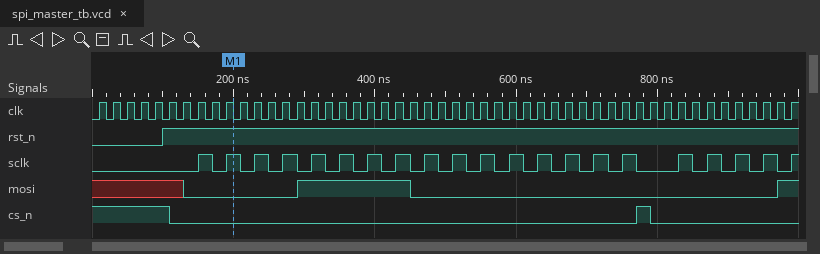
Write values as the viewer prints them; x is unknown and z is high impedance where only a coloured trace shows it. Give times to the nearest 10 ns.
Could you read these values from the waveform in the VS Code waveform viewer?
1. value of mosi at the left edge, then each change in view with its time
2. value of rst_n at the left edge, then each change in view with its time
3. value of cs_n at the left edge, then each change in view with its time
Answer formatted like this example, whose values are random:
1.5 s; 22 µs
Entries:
x, 0 at 130 ns, 1 at 290 ns, 0 at 450 ns, 1 at 970 ns; 0, 1 at 100 ns; 1, 0 at 110 ns, 1 at 770 ns, 0 at 790 ns
